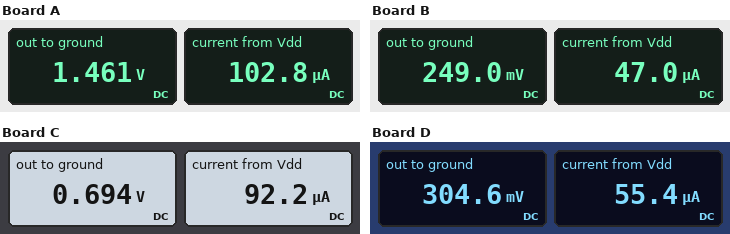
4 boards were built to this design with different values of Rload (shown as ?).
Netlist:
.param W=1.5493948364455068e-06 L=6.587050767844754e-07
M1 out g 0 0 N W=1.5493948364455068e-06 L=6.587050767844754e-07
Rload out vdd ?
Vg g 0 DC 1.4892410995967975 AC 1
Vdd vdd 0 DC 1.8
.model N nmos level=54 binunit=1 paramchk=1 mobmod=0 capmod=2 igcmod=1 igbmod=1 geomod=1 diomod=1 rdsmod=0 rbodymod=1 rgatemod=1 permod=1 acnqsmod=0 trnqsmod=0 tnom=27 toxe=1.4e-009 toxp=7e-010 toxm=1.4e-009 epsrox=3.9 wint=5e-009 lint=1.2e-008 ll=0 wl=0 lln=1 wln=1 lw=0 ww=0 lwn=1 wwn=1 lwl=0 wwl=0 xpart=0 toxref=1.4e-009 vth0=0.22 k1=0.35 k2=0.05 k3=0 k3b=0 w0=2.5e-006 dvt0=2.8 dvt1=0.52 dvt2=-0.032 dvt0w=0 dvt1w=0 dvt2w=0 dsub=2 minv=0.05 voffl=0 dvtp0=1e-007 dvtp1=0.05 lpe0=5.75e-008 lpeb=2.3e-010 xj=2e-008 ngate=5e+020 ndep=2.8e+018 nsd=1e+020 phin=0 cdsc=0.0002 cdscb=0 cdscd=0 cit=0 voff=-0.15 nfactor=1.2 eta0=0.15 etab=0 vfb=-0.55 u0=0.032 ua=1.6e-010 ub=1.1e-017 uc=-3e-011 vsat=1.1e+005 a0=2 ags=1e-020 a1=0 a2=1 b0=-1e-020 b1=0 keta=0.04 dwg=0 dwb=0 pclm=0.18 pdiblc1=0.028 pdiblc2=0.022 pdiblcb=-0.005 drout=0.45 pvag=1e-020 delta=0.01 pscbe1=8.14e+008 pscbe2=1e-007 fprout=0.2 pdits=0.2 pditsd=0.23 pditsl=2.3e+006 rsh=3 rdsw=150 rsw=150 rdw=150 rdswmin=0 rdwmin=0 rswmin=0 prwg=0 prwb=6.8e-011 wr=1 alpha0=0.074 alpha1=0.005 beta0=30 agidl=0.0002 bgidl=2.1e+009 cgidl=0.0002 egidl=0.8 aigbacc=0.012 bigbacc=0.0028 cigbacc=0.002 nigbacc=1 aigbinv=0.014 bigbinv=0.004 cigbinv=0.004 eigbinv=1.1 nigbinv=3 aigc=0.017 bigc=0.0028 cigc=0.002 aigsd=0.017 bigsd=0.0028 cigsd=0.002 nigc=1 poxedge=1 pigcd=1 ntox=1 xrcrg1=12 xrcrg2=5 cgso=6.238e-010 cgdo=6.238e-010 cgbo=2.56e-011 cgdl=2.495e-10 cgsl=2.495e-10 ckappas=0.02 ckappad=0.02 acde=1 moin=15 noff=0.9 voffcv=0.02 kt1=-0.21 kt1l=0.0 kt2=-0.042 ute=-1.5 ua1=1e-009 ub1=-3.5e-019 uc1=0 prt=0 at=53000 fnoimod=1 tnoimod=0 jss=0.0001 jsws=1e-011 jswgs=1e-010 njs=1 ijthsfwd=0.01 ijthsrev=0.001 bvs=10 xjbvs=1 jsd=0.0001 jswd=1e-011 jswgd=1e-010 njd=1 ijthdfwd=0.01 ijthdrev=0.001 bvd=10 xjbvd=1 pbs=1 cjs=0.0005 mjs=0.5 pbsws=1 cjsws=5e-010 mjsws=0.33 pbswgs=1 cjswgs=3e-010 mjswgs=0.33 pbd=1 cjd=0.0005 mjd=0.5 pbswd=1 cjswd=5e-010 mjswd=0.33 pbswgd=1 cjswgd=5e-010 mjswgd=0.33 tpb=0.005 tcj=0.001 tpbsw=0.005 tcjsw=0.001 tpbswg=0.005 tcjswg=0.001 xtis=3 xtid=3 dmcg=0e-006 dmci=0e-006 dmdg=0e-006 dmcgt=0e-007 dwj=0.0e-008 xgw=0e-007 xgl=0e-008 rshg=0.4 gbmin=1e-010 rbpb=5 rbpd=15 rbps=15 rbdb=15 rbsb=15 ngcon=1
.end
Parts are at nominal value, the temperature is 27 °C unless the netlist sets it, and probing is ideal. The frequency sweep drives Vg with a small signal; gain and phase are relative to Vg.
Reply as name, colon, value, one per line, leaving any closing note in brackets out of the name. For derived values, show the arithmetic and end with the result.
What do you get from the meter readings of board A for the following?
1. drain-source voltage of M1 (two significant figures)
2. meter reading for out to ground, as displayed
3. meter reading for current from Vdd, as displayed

drain-source voltage of M1: 1.461 V = 1.5 V
meter reading for out to ground, as displayed: 1.461 V
meter reading for current from Vdd, as displayed: 102.8 µA
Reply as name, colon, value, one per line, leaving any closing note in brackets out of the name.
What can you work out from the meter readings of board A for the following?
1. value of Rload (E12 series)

value of Rload: 3.3 kΩ
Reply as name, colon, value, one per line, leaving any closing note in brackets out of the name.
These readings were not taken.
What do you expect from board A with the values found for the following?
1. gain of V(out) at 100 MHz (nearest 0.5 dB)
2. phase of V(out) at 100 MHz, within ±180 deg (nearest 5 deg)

gain of V(out) at 100 MHz: -16.0 dB
phase of V(out) at 100 MHz, within ±180 deg: 170 deg
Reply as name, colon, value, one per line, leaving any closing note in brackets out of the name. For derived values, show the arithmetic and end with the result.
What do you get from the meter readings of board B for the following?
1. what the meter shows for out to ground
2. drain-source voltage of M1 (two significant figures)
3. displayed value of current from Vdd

what the meter shows for out to ground: 249.0 mV
drain-source voltage of M1: 249 mV = 250 mV
displayed value of current from Vdd: 47.0 µA
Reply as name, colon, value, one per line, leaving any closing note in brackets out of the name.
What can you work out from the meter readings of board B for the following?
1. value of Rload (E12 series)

value of Rload: 33 kΩ
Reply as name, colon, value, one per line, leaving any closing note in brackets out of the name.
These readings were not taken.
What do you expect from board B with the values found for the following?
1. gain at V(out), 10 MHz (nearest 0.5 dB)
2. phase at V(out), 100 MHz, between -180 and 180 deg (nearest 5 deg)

gain at V(out), 10 MHz: -33.0 dB
phase at V(out), 100 MHz, between -180 and 180 deg: 70 deg
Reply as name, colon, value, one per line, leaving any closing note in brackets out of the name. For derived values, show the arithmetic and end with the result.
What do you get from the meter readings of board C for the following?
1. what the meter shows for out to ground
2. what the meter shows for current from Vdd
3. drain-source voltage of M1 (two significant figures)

what the meter shows for out to ground: 0.694 V
what the meter shows for current from Vdd: 92.2 µA
drain-source voltage of M1: 694 mV = 690 mV
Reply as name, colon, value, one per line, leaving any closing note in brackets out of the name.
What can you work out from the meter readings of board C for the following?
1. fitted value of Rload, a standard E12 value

fitted value of Rload, a standard E12 value: 12 kΩ
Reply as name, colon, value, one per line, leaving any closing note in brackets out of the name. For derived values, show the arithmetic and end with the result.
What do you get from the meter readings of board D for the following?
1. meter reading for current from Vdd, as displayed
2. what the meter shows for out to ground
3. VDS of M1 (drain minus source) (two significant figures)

meter reading for current from Vdd, as displayed: 55.4 µA
what the meter shows for out to ground: 304.6 mV
VDS of M1 (drain minus source): 304.6 mV = 300 mV
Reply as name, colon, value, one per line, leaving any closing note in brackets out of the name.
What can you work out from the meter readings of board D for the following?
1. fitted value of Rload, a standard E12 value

fitted value of Rload, a standard E12 value: 27 kΩ
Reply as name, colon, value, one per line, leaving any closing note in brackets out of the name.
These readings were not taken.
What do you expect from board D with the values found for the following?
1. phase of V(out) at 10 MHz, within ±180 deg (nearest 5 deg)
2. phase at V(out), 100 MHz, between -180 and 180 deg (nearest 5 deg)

phase of V(out) at 10 MHz, within ±180 deg: 25 deg
phase at V(out), 100 MHz, between -180 and 180 deg: 75 deg
